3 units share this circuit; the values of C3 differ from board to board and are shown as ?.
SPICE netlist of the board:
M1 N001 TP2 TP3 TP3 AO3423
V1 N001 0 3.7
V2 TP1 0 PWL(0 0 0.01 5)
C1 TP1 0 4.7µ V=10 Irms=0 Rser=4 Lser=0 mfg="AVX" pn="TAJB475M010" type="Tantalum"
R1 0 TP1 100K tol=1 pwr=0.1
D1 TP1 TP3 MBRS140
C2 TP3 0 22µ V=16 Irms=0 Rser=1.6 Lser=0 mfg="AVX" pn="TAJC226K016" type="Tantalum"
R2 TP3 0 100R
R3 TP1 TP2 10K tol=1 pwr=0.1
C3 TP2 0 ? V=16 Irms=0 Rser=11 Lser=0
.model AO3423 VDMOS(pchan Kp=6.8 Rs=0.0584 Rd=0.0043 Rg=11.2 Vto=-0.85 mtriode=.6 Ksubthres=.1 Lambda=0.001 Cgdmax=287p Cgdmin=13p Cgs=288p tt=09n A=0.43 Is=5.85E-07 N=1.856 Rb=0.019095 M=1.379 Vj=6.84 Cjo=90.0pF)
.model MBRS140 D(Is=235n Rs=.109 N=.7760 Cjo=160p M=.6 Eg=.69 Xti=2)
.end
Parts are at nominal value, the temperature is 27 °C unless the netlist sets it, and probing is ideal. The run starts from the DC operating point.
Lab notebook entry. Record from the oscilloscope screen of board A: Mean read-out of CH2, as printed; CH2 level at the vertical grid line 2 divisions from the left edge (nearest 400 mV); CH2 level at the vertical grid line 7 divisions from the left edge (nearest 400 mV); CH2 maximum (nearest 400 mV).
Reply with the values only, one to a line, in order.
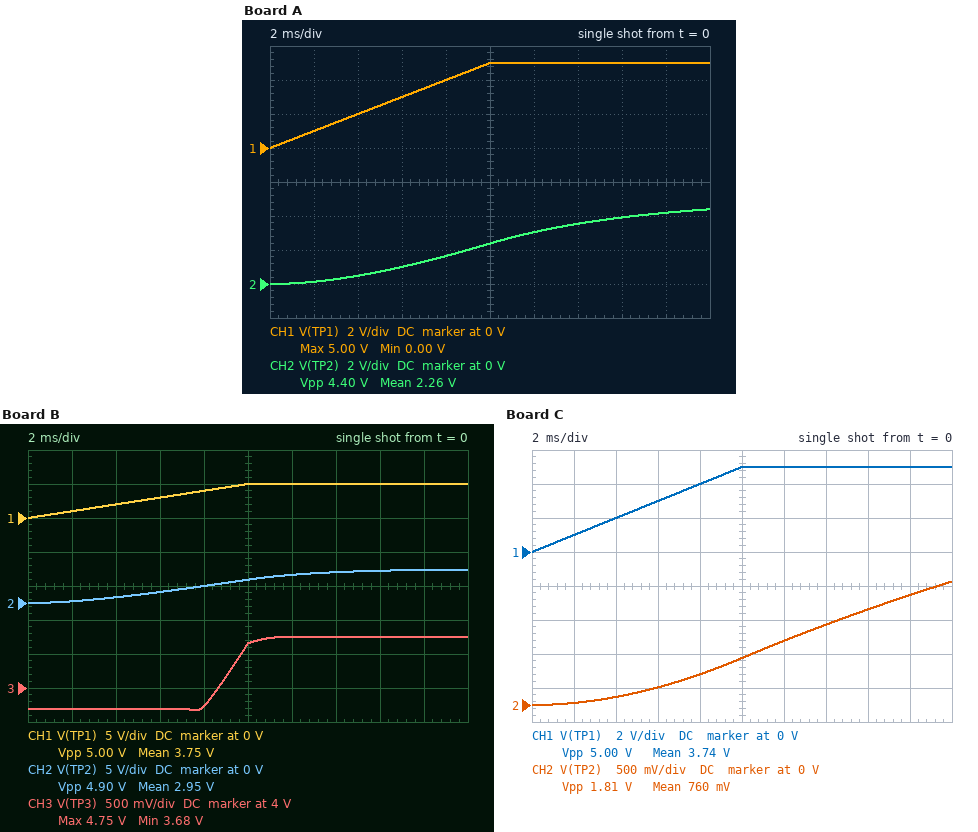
2.26 V
400 mV
3.6 V
4.4 V
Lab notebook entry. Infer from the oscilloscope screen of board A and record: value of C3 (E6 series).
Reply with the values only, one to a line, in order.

680 nF
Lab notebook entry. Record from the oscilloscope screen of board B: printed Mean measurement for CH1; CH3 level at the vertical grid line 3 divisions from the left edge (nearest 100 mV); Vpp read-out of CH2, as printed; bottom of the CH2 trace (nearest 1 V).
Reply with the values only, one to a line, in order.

3.75 V
3.7 V
4.90 V
0 V
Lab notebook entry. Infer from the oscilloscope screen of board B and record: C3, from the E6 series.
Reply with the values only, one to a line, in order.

330 nF
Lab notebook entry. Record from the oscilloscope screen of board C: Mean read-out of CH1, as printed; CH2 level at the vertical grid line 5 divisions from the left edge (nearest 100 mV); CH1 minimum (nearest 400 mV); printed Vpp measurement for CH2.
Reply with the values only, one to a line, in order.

3.74 V
700 mV
0 V
1.81 V
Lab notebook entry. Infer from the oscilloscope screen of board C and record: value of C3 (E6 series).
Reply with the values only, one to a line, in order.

3.3 µF
